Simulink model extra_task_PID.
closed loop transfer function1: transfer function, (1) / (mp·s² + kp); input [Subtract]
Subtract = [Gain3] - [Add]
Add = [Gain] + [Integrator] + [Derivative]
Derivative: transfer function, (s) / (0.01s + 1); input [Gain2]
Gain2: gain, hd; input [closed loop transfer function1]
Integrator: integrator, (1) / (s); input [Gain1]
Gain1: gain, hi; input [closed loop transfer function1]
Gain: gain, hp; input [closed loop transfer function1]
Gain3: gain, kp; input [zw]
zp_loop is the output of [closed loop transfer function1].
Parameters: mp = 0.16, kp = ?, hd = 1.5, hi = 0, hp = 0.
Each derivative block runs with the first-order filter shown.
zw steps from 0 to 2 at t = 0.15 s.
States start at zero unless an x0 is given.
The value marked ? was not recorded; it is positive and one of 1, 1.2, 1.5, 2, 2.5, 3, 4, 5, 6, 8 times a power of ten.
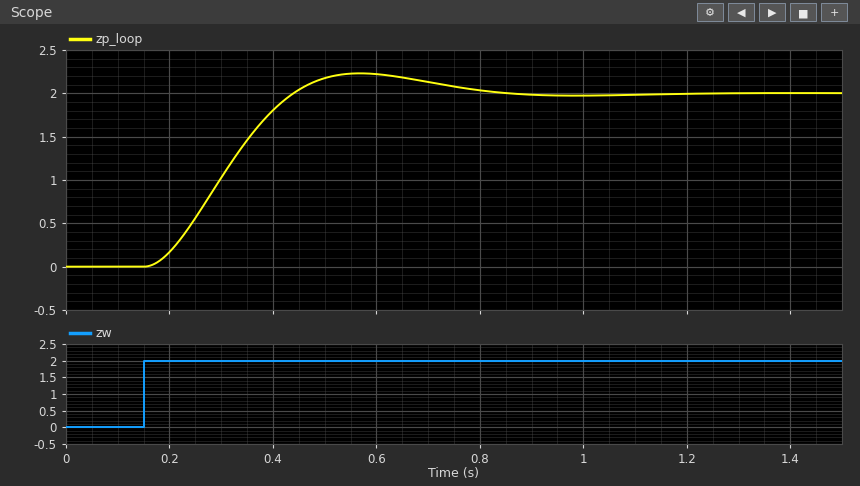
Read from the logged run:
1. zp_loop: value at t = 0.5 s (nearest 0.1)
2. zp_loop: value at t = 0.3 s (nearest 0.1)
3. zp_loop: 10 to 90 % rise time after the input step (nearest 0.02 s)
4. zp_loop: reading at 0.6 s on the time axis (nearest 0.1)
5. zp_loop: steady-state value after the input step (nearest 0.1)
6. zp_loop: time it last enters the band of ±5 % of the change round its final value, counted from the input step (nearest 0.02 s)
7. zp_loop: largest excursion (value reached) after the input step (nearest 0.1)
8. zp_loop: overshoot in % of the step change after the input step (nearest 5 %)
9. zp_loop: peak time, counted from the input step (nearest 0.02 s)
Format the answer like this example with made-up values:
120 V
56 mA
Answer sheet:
2.2
1.0
0.20 s
2.2
2.0
0.58 s
2.2
10 %
0.42 s
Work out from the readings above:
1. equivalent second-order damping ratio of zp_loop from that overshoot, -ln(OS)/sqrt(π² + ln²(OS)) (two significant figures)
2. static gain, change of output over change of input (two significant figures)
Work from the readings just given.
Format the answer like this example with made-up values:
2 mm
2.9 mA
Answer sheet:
0.59
1.0
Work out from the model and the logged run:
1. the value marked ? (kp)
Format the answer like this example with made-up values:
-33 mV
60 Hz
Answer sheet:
12
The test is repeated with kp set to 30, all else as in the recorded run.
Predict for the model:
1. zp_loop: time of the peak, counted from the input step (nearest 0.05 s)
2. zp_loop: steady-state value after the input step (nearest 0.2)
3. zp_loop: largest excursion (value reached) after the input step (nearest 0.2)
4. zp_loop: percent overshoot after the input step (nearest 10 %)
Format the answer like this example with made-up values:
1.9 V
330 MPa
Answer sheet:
0.25 s
2.0
2.6
30 %
